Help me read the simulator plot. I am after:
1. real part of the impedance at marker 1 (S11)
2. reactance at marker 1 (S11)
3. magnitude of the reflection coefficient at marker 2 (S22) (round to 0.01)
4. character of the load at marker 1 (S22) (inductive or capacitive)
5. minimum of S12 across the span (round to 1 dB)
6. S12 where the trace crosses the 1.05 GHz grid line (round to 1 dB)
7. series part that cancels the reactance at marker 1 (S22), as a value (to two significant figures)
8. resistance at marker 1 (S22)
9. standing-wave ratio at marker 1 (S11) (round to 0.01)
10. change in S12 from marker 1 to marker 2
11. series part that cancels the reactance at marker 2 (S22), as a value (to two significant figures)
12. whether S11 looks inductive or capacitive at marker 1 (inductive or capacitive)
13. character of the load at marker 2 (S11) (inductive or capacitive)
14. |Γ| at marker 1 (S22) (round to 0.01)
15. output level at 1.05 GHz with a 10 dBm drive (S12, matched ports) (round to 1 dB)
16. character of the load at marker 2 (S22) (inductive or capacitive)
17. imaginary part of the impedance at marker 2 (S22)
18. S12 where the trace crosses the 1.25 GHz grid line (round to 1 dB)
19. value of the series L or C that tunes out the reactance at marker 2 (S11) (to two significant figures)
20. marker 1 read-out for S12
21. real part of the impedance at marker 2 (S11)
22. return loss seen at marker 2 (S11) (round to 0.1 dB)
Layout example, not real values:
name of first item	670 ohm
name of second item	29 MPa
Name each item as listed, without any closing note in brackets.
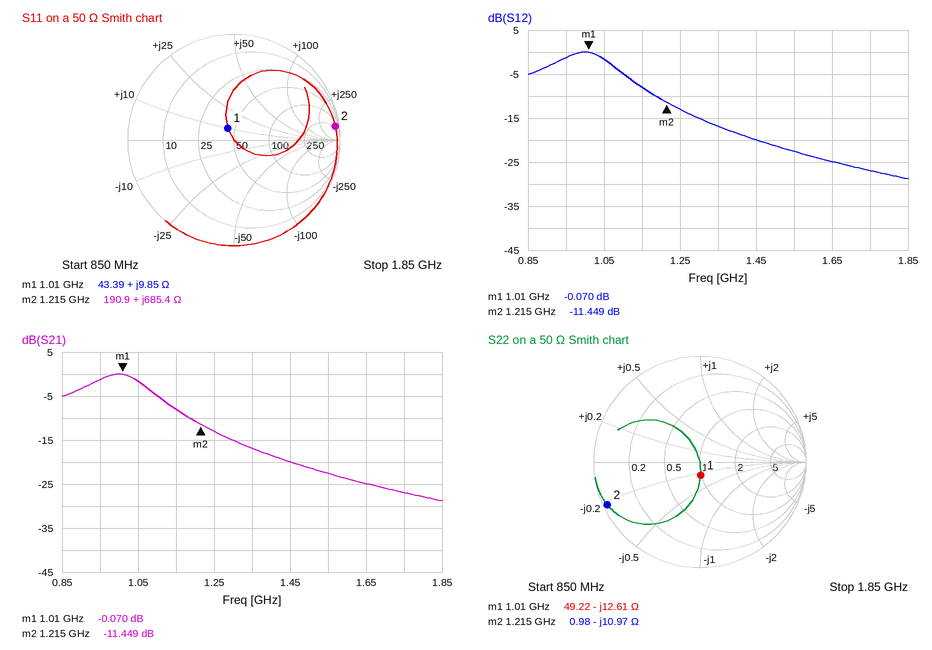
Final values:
real part of the impedance at marker 1	43.39 Ω
reactance at marker 1	+9.85 Ω
magnitude of the reflection coefficient at marker 2 (S22)	0.96
character of the load at marker 1 (S22)	capacitive
minimum of S12 across the span	-29 dB
S12 where the trace crosses the 1.05 GHz grid line	-2 dB
series part that cancels the reactance at marker 1 (S22), as a value	2.0 nH
resistance at marker 1	49.22 Ω
standing-wave ratio at marker 1 (S11)	1.29
change in S12 from marker 1 to marker 2	-11.379 dB
series part that cancels the reactance at marker 2 (S22), as a value	1.4 nH
whether S11 looks inductive or capacitive at marker 1	inductive
character of the load at marker 2 (S11)	inductive
|Γ| at marker 1 (S22)	0.13
output level at 1.05 GHz with a 10 dBm drive (S12, matched ports)	8 dBm
character of the load at marker 2 (S22)	capacitive
imaginary part of the impedance at marker 2	-10.97 Ω
S12 where the trace crosses the 1.25 GHz grid line	-13 dB
value of the series L or C that tunes out the reactance at marker 2 (S11)	190 fF
marker 1 read-out for S12	-0.070 dB
real part of the impedance at marker 2	190.9 Ω
return loss seen at marker 2 (S11)	0.3 dB
